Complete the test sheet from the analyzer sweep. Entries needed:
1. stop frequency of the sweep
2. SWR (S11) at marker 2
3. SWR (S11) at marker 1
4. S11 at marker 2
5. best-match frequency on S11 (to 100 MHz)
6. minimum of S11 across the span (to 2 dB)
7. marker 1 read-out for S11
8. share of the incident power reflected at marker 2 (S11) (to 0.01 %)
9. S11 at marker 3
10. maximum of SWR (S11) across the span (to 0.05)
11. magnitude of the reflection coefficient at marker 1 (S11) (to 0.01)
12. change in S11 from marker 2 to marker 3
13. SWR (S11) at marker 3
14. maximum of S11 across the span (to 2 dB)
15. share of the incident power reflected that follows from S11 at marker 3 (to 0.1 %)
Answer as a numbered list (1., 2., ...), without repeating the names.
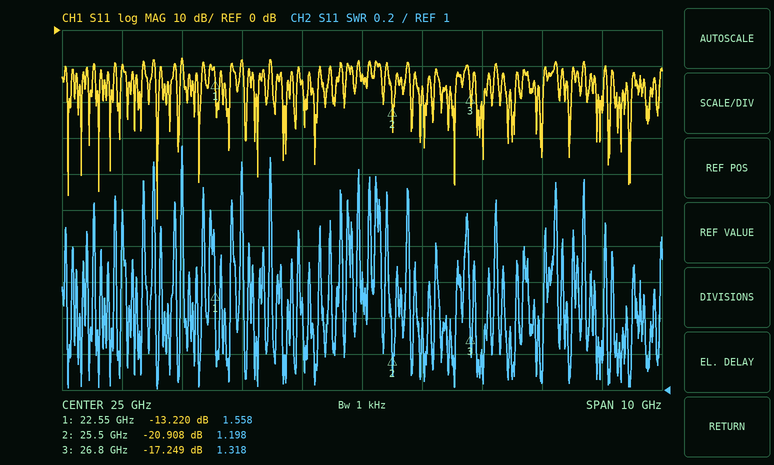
1. 30 GHz
2. 1.198
3. 1.558
4. -20.908 dB
5. 21.6 GHz
6. -52 dB
7. -13.220 dB
8. 0.81 %
9. -17.249 dB
10. 2.35
11. 0.22
12. 3.659 dB
13. 1.318
14. -8 dB
15. 1.9 %
